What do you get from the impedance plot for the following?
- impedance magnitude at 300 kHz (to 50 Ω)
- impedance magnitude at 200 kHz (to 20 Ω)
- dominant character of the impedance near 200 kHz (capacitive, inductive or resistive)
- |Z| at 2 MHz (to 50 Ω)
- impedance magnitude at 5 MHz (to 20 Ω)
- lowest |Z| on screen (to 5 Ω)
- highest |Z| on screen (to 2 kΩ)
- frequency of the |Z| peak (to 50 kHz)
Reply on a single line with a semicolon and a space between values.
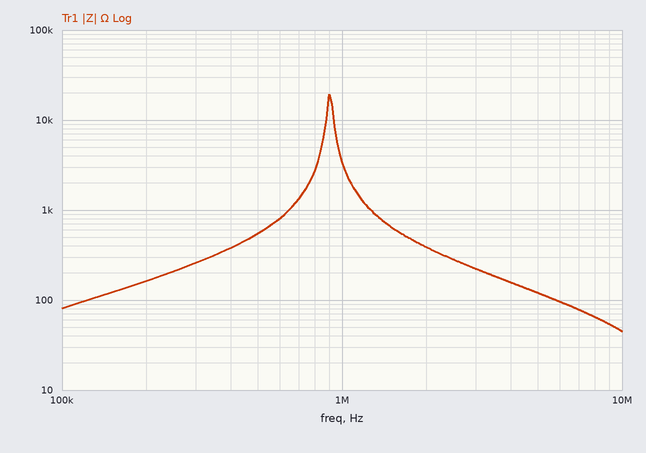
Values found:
250 Ω; 160 Ω; inductive; 400 Ω; 120 Ω; 45 Ω; 20 kΩ; 900 kHz
